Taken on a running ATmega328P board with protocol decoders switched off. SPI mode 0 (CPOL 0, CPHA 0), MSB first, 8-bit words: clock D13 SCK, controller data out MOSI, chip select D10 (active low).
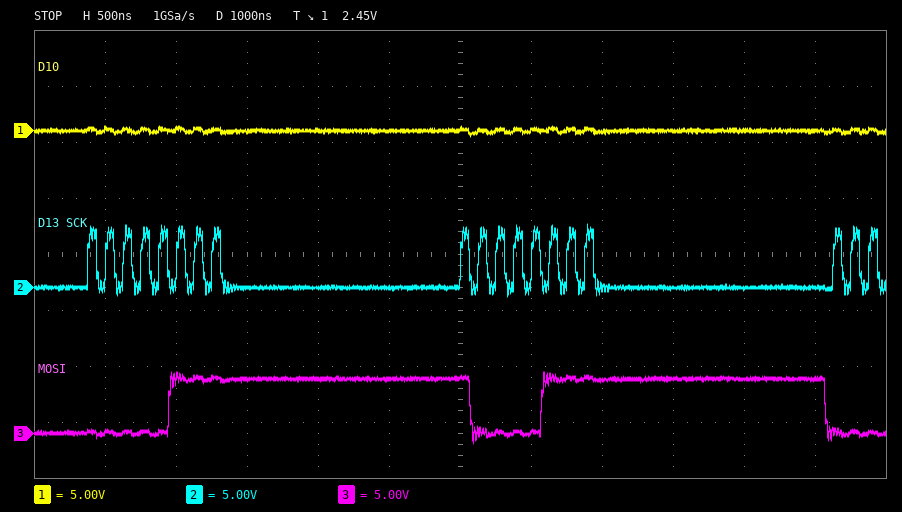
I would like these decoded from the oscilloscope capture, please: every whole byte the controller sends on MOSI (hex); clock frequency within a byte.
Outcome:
07 87
8 MHz
